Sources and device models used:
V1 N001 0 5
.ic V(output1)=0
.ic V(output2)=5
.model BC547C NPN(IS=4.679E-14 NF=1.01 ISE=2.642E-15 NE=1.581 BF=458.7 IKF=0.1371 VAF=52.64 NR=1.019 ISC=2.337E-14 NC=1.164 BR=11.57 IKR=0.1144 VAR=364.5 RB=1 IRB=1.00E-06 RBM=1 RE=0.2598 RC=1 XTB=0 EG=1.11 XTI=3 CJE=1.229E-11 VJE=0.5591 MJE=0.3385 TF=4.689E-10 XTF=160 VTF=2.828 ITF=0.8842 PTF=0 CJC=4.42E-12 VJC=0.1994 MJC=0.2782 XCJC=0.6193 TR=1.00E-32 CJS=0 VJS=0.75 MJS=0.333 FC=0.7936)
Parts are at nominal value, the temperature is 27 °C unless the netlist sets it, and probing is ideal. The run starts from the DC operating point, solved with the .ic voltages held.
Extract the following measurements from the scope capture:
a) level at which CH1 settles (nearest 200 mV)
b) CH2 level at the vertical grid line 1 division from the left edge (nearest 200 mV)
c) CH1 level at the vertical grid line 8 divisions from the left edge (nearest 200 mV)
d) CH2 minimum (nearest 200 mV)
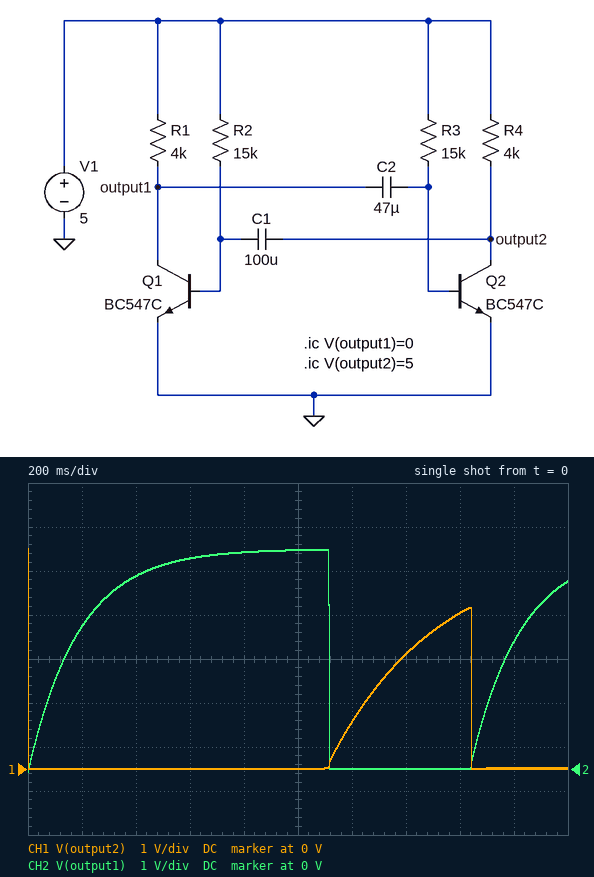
0 V
3.2 V
3.6 V
0 V
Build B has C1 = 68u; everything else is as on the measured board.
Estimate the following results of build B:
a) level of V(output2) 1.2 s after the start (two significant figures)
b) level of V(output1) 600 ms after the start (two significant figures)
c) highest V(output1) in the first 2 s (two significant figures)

4.0 V
4.8 V
4.9 V
